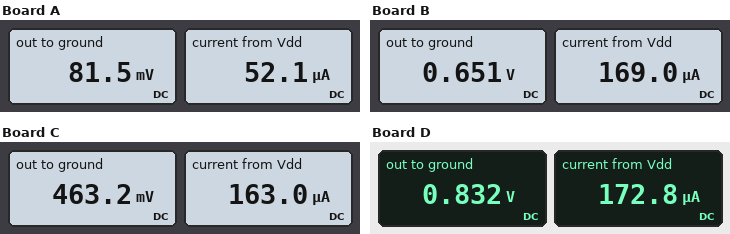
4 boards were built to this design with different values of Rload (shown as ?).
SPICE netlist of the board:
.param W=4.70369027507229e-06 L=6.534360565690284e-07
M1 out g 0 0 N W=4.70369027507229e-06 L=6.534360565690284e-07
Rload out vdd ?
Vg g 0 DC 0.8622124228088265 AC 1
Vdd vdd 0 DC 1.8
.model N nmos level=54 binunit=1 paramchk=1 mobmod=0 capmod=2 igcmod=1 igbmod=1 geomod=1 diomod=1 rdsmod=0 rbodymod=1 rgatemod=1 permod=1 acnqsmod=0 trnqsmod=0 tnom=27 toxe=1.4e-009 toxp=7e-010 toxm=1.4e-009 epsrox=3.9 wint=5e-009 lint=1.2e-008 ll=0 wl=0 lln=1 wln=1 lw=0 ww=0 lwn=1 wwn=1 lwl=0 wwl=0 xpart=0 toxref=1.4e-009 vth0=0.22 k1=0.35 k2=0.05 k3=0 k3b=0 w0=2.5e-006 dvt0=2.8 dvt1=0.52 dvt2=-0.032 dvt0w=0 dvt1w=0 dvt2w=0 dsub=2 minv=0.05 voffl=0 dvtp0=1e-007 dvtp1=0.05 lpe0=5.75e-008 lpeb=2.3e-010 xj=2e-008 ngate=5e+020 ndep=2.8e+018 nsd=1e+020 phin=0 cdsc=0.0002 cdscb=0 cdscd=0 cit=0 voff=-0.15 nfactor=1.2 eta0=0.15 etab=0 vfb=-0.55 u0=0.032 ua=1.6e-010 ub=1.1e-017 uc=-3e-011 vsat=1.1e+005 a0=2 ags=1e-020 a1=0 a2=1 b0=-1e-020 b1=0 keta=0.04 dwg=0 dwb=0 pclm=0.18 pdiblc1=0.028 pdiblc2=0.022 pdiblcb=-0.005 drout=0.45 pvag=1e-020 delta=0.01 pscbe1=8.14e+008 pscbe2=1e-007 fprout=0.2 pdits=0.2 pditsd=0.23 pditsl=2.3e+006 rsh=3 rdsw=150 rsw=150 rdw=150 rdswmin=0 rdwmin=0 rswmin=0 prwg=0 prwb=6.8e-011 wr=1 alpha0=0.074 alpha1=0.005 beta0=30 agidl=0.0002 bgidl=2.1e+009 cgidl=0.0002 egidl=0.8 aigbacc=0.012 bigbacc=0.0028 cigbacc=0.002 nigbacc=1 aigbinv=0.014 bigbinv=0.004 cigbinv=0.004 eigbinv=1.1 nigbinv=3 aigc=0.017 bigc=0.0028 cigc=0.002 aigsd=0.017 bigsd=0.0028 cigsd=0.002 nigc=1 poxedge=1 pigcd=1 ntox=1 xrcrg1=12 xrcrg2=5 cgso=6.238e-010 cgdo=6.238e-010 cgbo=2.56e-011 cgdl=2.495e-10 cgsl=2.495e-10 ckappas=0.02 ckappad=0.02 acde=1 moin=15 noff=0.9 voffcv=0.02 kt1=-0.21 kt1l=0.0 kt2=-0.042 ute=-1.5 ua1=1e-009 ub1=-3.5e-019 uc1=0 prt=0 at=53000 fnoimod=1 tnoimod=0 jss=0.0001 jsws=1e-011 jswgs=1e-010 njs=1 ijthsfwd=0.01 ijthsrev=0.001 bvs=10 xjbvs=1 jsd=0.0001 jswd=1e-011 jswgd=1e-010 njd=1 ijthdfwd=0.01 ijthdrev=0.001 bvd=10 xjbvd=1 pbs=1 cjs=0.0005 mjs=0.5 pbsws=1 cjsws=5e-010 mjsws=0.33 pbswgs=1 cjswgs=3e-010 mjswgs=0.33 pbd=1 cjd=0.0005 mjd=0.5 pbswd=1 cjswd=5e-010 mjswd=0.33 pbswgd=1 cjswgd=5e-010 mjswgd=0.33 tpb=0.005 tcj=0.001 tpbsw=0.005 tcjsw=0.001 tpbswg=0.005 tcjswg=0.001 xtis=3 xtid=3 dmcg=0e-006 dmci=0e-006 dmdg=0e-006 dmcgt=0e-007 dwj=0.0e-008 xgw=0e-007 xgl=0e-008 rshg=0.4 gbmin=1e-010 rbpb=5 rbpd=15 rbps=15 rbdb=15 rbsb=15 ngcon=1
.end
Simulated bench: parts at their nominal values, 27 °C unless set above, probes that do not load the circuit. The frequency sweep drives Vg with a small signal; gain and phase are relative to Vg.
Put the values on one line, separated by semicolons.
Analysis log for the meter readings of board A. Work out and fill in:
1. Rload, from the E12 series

33 kΩ
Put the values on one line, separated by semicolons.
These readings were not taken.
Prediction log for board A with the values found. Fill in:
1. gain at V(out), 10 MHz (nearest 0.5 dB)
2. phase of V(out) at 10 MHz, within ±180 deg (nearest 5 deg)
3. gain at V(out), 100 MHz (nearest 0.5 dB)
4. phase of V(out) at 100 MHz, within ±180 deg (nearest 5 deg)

-29.5 dB; 170 deg; -23.0 dB; 115 deg
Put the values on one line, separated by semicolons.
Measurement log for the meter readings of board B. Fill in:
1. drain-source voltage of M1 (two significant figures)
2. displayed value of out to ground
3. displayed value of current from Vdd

650 mV; 0.651 V; 169.0 µA
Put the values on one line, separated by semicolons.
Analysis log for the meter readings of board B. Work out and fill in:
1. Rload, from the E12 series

6.8 kΩ
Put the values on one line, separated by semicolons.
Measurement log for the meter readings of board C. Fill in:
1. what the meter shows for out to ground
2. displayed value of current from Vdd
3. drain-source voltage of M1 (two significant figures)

463.2 mV; 163.0 µA; 460 mV
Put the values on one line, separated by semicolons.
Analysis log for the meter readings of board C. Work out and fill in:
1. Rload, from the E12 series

8.2 kΩ
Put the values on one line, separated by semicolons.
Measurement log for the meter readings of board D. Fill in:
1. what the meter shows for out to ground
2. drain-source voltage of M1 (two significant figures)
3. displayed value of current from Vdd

0.832 V; 830 mV; 172.8 µA
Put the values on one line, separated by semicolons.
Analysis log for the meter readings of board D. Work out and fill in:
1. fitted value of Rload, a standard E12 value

5.6 kΩ
